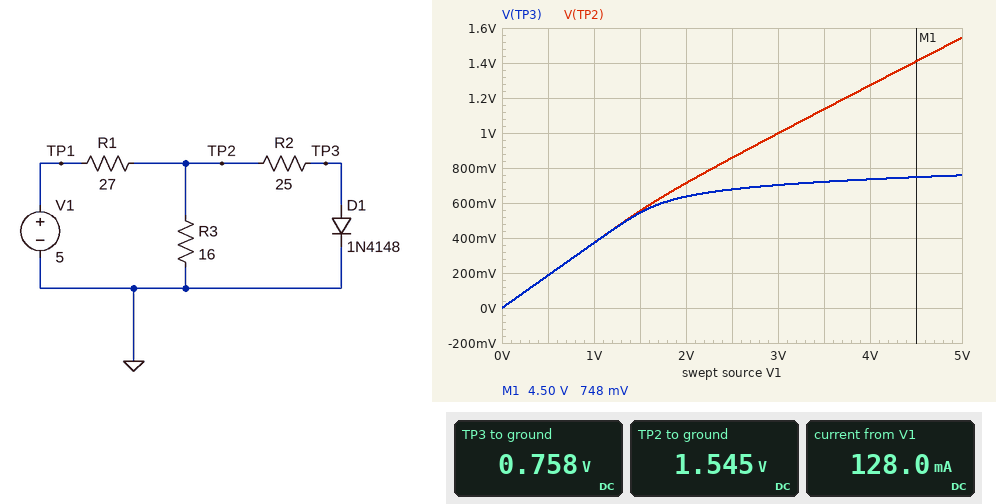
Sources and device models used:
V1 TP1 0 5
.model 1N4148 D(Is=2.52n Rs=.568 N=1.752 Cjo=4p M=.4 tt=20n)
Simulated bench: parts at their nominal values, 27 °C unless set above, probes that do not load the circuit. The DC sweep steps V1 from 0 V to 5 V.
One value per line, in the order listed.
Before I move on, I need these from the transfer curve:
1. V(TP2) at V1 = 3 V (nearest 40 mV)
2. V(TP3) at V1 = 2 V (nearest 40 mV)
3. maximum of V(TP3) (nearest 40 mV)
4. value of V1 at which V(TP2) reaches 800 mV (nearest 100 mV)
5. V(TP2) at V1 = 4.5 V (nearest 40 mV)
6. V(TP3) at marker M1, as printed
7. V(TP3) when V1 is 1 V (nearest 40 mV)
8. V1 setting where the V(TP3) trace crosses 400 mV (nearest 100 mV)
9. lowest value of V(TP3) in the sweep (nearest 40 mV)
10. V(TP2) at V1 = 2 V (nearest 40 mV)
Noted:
1.00 V
640 mV
760 mV
2.3 V
1.40 V
748 mV
360 mV
1.1 V
0 V
720 mV
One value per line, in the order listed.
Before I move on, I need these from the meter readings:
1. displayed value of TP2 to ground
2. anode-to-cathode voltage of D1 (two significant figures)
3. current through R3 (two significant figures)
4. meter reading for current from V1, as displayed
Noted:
1.545 V
760 mV
97 mA
128.0 mA
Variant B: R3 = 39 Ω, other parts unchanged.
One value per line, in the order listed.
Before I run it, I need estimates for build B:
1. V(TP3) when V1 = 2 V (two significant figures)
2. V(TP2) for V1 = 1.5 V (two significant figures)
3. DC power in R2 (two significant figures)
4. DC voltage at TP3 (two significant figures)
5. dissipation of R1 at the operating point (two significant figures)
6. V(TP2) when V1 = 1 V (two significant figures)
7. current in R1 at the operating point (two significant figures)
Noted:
700 mV
800 mV
70 mW
790 mV
310 mW
580 mV
110 mA
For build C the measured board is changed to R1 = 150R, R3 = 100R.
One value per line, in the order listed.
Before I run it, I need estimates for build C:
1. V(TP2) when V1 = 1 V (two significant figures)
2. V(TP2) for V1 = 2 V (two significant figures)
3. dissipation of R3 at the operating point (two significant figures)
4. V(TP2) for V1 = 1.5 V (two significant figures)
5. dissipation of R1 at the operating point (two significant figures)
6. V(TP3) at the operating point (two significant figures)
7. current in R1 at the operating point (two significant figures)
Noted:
400 mV
670 mV
12 mW
570 mV
100 mW
720 mV
26 mA
